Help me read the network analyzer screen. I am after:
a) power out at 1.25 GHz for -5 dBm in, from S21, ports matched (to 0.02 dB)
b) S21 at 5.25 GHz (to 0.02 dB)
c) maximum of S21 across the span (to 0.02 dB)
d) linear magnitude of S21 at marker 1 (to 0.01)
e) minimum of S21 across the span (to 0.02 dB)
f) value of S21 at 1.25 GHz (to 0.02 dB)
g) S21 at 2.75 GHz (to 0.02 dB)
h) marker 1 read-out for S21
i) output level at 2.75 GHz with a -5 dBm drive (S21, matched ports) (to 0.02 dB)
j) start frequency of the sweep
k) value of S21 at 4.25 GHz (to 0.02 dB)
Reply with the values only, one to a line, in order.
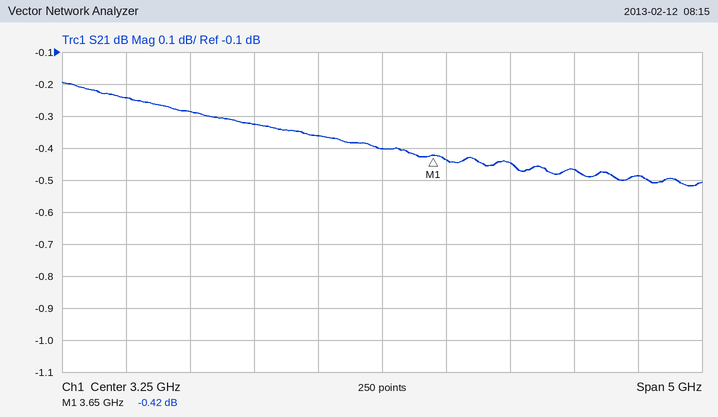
-5.24 dBm
-0.48 dB
-0.20 dB
0.95
-0.52 dB
-0.24 dB
-0.36 dB
-0.42 dB
-5.36 dBm
750 MHz
-0.44 dB
